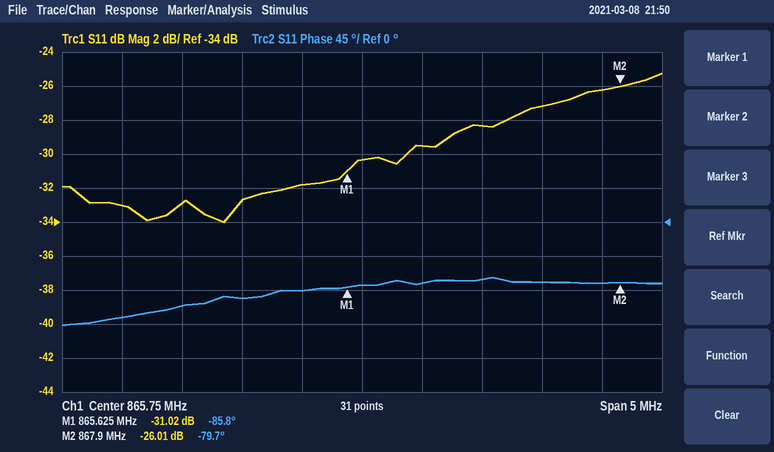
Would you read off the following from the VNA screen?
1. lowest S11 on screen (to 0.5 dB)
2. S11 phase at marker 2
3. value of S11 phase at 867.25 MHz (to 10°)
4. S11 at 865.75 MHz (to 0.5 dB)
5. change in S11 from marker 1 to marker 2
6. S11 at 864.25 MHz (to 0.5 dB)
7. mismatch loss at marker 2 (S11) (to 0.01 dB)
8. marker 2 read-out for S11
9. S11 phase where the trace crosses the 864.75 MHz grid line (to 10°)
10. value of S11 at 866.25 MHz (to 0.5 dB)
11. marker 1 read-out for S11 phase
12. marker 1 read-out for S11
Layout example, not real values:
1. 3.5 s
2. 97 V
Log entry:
1. -34.0 dB
2. -79.7°
3. -80°
4. -30.5 dB
5. 5.01 dB
6. -33.0 dB
7. 0.01 dB
8. -26.01 dB
9. -100°
10. -29.5 dB
11. -85.8°
12. -31.02 dB
